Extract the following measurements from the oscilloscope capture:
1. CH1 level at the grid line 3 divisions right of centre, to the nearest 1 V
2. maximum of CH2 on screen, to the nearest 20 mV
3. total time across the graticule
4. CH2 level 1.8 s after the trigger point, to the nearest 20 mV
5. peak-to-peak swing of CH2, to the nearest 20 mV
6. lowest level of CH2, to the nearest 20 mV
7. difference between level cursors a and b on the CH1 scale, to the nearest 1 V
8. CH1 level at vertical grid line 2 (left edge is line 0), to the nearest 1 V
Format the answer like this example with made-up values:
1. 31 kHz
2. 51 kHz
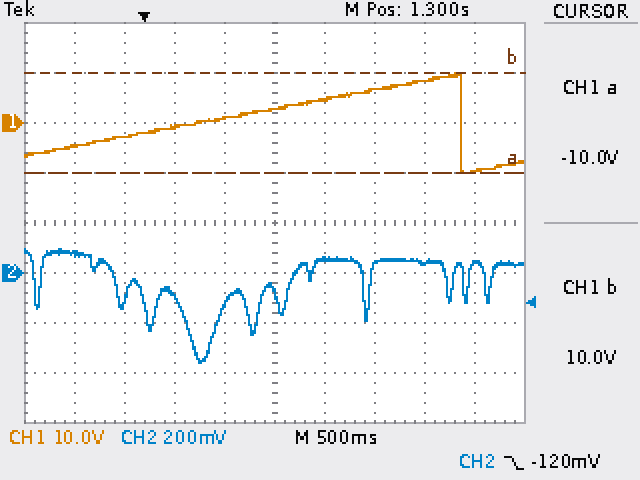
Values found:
1. 8 V
2. 100 mV
3. 5 s
4. 60 mV
5. 460 mV
6. -360 mV
7. 20 V
8. -3 V
